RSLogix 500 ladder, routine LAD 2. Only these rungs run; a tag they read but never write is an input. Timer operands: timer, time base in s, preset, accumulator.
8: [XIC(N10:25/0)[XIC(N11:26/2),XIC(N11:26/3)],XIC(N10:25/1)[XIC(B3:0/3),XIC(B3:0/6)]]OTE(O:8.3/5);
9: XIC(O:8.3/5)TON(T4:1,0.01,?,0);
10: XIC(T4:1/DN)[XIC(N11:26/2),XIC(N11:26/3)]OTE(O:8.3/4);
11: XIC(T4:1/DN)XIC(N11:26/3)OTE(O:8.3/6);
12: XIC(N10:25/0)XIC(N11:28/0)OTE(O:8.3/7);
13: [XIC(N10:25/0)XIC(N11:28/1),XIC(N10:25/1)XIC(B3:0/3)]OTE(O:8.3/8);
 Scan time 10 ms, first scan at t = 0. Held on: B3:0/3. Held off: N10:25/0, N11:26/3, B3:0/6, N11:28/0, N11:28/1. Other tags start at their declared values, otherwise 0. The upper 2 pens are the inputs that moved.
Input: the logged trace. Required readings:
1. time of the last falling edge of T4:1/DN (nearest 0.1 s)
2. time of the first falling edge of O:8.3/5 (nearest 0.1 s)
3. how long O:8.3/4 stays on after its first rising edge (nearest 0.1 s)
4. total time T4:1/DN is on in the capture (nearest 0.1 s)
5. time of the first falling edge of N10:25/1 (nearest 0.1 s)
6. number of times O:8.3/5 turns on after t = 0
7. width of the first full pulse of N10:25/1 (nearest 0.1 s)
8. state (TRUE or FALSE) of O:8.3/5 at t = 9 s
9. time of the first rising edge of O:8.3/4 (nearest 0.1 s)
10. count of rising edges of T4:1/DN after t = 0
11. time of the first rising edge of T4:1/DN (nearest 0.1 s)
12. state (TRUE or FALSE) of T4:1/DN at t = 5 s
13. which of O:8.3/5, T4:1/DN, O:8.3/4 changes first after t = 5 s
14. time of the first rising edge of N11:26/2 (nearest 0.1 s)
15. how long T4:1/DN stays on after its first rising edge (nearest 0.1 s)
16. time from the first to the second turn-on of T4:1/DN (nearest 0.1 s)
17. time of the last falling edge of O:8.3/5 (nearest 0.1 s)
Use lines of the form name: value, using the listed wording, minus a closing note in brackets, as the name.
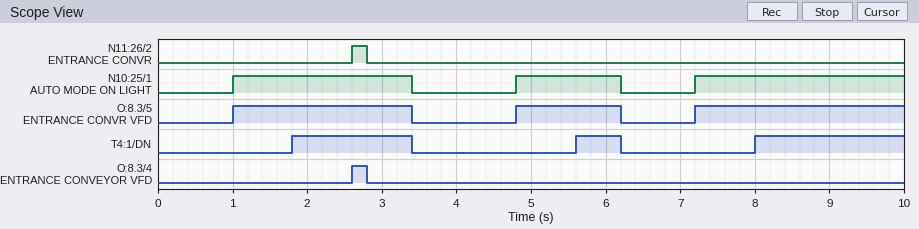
time of the last falling edge of T4:1/DN: 6.2 s
time of the first falling edge of O:8.3/5: 3.4 s
how long O:8.3/4 stays on after its first rising edge: 0.2 s
total time T4:1/DN is on in the capture: 4.2 s
time of the first falling edge of N10:25/1: 3.4 s
number of times O:8.3/5 turns on after t = 0: 3
width of the first full pulse of N10:25/1: 2.4 s
state (TRUE or FALSE) of O:8.3/5 at t = 9 s: TRUE
time of the first rising edge of O:8.3/4: 2.6 s
count of rising edges of T4:1/DN after t = 0: 3
time of the first rising edge of T4:1/DN: 1.8 s
state (TRUE or FALSE) of T4:1/DN at t = 5 s: FALSE
which of O:8.3/5, T4:1/DN, O:8.3/4 changes first after t = 5 s: T4:1/DN
time of the first rising edge of N11:26/2: 2.6 s
how long T4:1/DN stays on after its first rising edge: 1.6 s
time from the first to the second turn-on of T4:1/DN: 3.8 s
time of the last falling edge of O:8.3/5: 6.2 s
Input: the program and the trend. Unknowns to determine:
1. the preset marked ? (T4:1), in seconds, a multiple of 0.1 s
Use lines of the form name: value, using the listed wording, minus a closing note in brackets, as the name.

the preset marked ? (T4:1), in seconds, a multiple of 0.1 s: 0.8 s
